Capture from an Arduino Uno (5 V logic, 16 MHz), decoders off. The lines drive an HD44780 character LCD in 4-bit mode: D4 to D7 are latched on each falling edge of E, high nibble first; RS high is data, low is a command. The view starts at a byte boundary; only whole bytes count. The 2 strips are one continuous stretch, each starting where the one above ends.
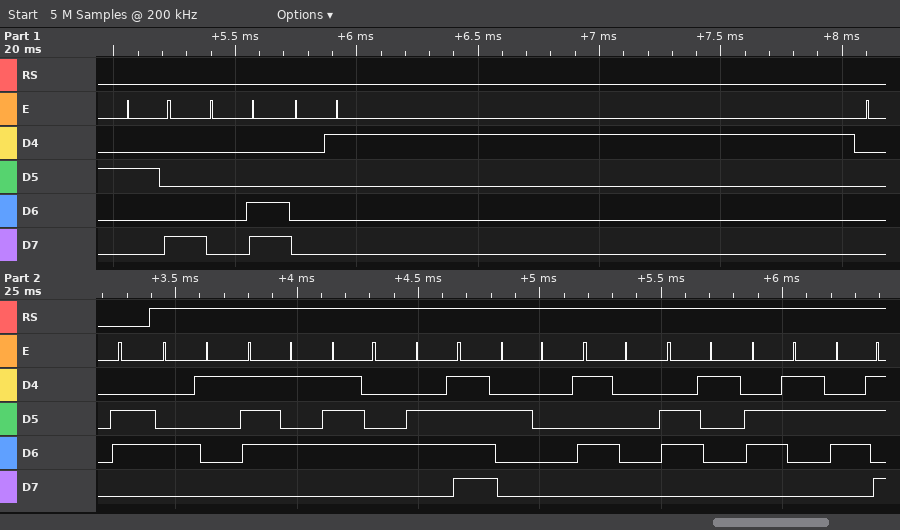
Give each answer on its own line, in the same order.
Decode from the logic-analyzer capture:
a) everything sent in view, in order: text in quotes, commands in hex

0x28 0x0C 0x01 0x06 "Auto Pack"
